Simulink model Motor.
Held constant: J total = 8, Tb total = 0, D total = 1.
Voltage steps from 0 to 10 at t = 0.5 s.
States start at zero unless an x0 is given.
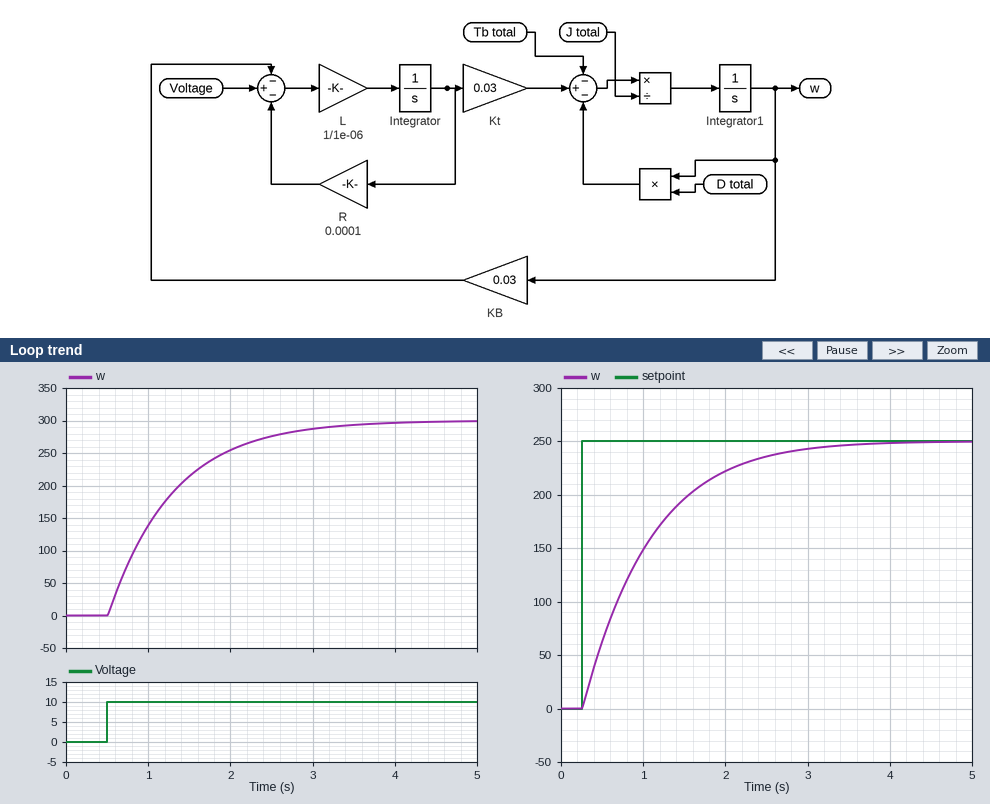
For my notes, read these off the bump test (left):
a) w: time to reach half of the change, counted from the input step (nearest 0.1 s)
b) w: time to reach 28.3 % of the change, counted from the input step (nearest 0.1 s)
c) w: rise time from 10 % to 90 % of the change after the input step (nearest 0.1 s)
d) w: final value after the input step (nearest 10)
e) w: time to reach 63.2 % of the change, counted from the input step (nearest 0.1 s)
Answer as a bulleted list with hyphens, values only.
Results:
- 0.6 s
- 0.3 s
- 1.7 s
- 300
- 0.8 s
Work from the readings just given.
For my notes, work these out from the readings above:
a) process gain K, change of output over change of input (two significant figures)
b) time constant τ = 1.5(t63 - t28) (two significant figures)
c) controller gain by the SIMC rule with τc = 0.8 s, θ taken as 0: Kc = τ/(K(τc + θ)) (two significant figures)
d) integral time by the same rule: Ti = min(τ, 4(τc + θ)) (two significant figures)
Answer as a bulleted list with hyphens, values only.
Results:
- 30
- 0.75 s
- 0.031
- 0.75 s
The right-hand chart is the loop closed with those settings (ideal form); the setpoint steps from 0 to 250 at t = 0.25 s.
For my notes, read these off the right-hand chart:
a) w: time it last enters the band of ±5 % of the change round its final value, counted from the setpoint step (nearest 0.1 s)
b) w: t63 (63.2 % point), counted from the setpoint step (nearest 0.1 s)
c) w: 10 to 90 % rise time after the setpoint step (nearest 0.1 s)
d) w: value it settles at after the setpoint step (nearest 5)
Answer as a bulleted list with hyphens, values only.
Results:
- 2.3 s
- 0.8 s
- 1.7 s
- 250
